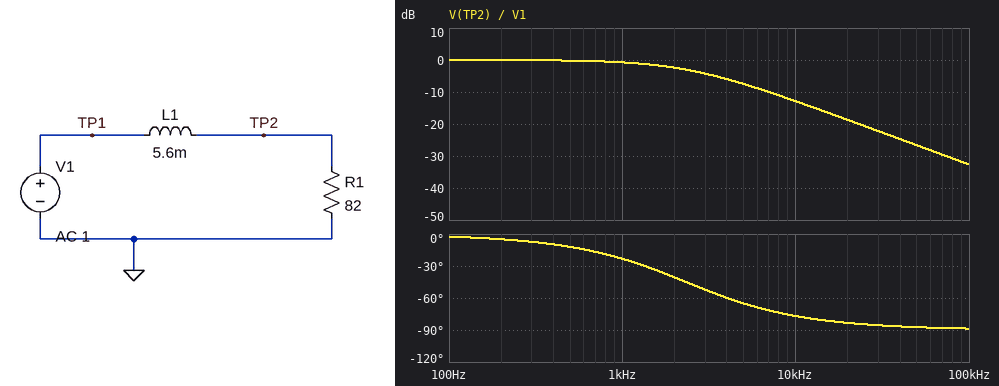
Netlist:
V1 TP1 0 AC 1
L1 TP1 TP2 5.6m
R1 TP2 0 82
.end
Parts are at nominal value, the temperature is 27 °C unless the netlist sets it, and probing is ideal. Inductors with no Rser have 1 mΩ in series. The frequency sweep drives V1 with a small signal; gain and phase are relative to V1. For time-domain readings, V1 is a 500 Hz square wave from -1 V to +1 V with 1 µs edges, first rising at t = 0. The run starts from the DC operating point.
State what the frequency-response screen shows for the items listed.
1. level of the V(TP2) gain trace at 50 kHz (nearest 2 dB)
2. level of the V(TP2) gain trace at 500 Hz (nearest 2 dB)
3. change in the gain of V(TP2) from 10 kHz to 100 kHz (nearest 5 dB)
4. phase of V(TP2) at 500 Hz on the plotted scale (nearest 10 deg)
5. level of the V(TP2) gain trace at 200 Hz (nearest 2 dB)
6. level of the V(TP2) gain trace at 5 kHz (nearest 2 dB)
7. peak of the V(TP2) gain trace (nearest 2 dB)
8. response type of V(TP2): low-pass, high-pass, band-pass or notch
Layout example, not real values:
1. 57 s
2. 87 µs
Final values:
1. -26 dB
2. 0 dB
3. -20 dB
4. -10 deg
5. 0 dB
6. -8 dB
7. 0 dB
8. low-pass
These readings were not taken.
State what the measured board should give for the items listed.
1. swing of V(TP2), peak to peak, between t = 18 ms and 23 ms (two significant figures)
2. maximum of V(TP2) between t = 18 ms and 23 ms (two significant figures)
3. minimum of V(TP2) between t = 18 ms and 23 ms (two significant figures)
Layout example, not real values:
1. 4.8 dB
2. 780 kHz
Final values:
1. 2.0 V
2. 1.0 V
3. -1.0 V
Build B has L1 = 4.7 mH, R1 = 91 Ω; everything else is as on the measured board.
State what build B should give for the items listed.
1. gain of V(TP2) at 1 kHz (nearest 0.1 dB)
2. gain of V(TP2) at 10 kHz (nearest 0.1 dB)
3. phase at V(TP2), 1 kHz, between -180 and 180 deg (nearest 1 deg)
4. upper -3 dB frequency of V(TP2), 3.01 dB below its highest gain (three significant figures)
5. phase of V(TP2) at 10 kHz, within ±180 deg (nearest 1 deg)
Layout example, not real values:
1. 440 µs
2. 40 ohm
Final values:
1. -0.4 dB
2. -10.6 dB
3. -18 deg
4. 3.08 kHz
5. -73 deg
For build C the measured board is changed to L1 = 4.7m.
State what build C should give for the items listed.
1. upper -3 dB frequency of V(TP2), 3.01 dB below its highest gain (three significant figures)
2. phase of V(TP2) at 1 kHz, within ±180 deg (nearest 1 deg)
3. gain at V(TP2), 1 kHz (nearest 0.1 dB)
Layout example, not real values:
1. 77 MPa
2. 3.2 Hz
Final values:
1. 2.78 kHz
2. -20 deg
3. -0.5 dB
